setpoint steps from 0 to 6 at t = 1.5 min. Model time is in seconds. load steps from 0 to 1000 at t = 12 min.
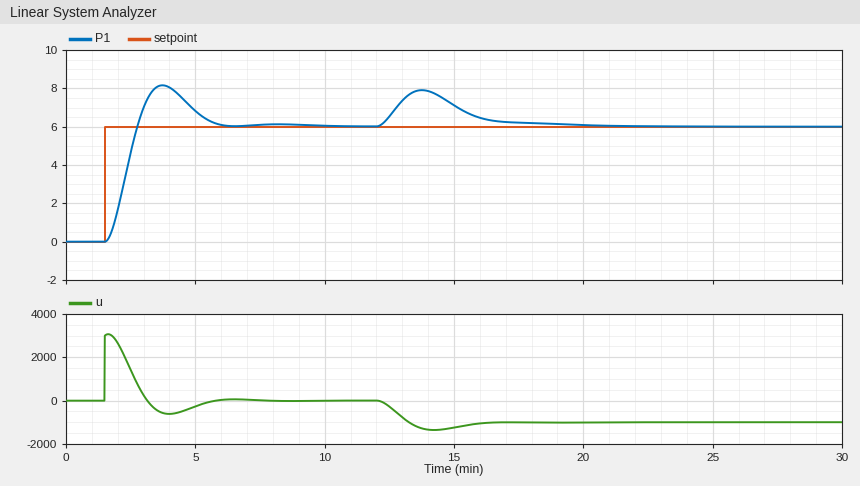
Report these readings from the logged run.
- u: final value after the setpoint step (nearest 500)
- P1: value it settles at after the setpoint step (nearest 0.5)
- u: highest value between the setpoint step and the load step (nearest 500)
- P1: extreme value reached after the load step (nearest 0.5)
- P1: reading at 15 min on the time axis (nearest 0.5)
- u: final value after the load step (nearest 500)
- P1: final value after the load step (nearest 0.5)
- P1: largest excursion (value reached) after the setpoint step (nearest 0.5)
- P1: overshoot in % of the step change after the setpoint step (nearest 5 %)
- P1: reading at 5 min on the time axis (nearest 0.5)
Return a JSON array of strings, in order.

["0", "6.0", "3000", "8.0", "7.0", "-1000", "6.0", "8.0", "35 %", "7.0"]
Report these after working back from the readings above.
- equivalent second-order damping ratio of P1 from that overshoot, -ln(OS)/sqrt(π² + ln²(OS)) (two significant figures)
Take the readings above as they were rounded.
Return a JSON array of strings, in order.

["0.32"]
